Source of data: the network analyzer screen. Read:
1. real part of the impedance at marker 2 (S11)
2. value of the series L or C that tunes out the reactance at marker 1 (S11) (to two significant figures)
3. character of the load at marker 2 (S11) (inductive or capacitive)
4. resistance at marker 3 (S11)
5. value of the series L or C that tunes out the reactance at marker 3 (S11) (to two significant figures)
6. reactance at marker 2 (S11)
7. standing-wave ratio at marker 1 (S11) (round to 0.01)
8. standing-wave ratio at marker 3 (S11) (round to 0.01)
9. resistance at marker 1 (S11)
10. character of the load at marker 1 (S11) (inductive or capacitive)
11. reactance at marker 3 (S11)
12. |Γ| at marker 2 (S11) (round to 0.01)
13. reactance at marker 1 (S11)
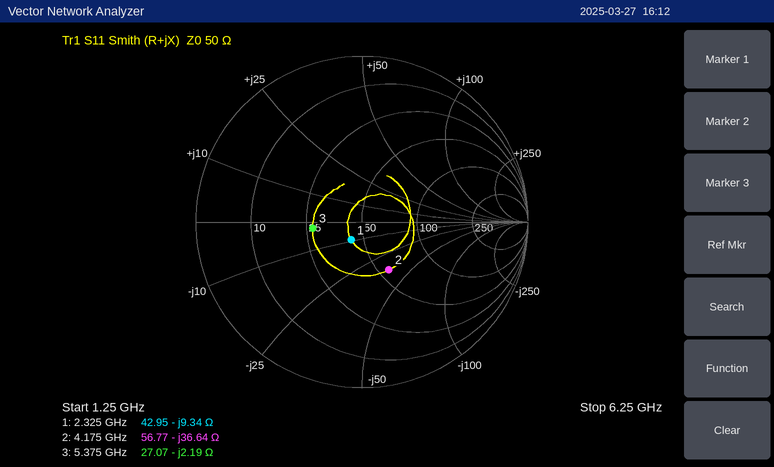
56.77 Ω
640 pH
capacitive
27.07 Ω
65 pH
-36.64 Ω
1.29
1.85
42.95 Ω
capacitive
-2.19 Ω
0.33
-9.34 Ω
